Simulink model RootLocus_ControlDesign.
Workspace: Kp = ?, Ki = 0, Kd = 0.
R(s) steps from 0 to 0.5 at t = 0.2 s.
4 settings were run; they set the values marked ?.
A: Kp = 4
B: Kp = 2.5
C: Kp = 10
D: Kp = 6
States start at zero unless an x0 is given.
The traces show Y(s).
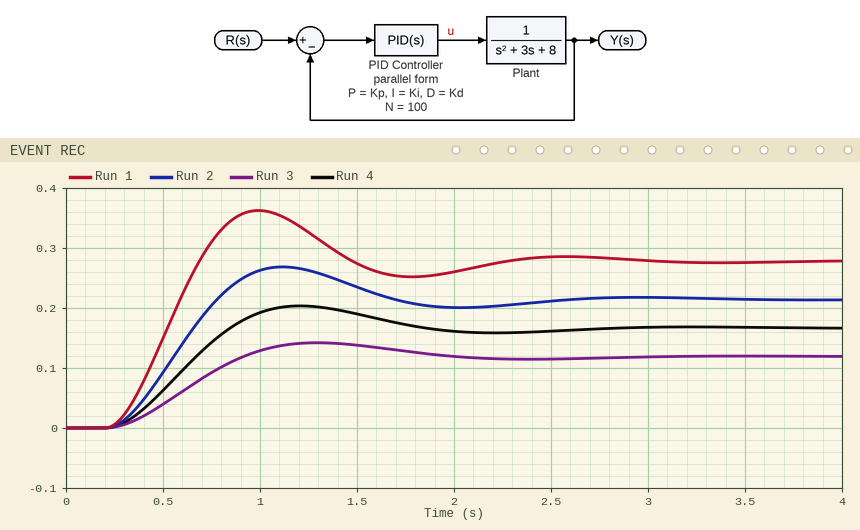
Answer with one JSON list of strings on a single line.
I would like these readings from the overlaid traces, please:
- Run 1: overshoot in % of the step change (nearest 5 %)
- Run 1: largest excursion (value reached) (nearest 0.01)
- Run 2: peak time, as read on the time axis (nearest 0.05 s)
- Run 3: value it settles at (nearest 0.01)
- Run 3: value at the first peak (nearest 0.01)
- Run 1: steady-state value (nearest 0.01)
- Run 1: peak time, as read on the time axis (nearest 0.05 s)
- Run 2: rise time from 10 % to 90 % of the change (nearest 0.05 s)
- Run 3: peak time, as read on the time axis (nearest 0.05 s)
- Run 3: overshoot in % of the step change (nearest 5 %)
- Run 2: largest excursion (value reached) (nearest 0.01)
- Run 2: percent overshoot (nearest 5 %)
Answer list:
["30 %", "0.36", "1.10 s", "0.12", "0.14", "0.28", "1.00 s", "0.40 s", "1.30 s", "20 %", "0.27", "25 %"]
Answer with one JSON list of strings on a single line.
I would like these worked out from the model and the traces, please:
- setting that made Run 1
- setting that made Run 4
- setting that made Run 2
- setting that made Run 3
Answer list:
["C", "A", "D", "B"]
